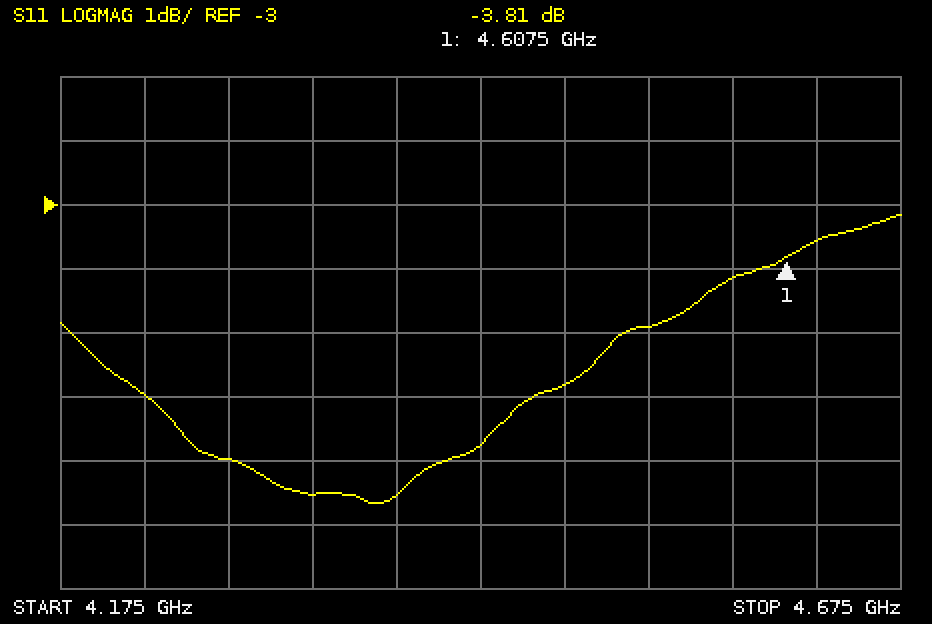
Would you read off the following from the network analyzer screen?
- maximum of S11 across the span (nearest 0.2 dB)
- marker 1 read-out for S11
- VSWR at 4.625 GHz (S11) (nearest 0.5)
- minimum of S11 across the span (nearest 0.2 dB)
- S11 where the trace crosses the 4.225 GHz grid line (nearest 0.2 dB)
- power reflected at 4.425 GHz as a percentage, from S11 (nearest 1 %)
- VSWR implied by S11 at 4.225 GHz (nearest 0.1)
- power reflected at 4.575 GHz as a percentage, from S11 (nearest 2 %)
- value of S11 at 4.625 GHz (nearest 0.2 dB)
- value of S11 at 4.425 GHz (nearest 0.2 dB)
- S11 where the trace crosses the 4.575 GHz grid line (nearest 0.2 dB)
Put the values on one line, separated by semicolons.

-3.2 dB; -3.81 dB; 5.0; -7.6 dB; -6.0 dB; 21 %; 3.0; 38 %; -3.6 dB; -6.8 dB; -4.2 dB
